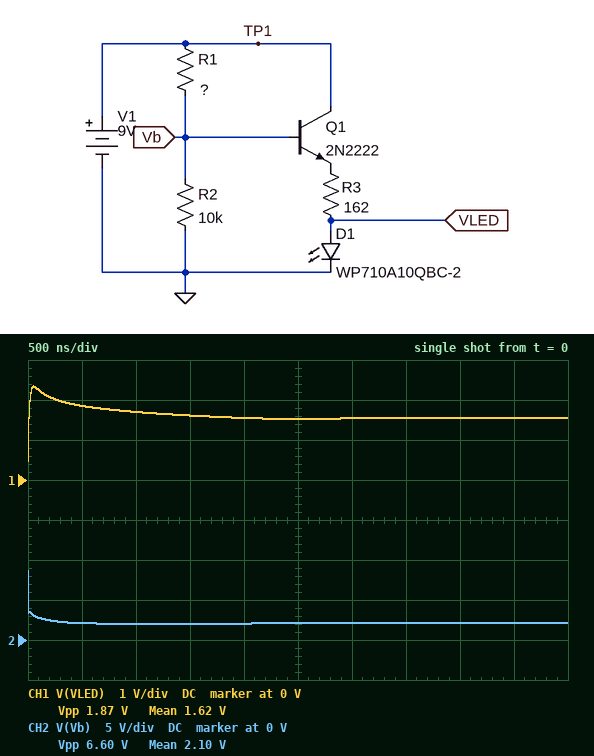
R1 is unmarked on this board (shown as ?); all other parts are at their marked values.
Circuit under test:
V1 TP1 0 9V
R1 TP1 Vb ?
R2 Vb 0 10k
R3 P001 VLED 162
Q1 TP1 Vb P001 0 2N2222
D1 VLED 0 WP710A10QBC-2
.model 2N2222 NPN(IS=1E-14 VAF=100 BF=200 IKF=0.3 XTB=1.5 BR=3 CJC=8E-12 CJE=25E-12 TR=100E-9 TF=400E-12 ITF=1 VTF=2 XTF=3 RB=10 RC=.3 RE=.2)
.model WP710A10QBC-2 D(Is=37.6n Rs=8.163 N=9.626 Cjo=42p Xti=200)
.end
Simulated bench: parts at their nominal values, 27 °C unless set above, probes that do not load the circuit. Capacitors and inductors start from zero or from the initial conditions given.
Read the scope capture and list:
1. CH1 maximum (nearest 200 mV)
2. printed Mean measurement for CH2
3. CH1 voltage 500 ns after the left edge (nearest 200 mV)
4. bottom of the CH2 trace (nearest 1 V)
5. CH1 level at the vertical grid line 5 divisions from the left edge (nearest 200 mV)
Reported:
2.4 V
2.10 V
1.8 V
2 V
1.6 V
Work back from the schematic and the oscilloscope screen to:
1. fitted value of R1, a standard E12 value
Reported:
33 kΩ
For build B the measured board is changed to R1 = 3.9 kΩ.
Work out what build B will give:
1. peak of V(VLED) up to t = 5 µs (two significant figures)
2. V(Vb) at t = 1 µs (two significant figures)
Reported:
3.3 V
6.3 V
